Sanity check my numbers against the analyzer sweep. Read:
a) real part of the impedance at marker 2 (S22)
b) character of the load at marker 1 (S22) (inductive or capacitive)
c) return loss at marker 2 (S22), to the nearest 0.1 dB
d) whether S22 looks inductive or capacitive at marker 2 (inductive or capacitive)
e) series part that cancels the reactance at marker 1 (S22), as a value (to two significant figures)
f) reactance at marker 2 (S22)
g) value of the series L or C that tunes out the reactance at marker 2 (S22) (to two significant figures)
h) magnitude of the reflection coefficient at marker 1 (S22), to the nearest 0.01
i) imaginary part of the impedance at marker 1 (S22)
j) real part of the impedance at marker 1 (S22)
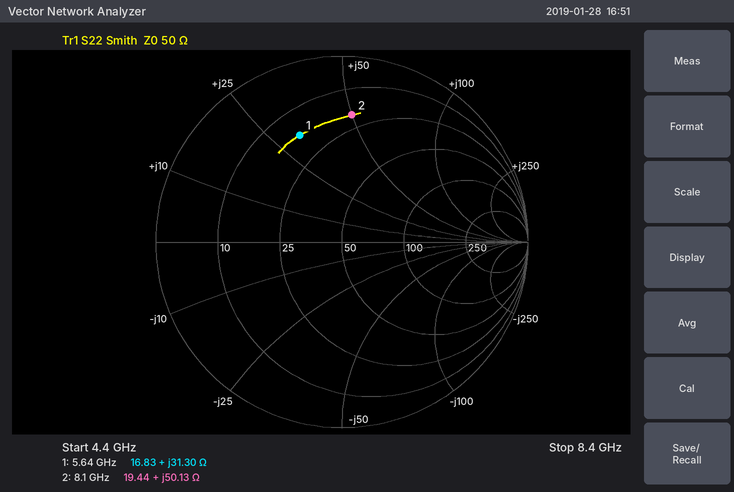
19.44 Ω
inductive
3.3 dB
inductive
900 fF
+50.13 Ω
390 fF
0.62
+31.30 Ω
16.83 Ω
